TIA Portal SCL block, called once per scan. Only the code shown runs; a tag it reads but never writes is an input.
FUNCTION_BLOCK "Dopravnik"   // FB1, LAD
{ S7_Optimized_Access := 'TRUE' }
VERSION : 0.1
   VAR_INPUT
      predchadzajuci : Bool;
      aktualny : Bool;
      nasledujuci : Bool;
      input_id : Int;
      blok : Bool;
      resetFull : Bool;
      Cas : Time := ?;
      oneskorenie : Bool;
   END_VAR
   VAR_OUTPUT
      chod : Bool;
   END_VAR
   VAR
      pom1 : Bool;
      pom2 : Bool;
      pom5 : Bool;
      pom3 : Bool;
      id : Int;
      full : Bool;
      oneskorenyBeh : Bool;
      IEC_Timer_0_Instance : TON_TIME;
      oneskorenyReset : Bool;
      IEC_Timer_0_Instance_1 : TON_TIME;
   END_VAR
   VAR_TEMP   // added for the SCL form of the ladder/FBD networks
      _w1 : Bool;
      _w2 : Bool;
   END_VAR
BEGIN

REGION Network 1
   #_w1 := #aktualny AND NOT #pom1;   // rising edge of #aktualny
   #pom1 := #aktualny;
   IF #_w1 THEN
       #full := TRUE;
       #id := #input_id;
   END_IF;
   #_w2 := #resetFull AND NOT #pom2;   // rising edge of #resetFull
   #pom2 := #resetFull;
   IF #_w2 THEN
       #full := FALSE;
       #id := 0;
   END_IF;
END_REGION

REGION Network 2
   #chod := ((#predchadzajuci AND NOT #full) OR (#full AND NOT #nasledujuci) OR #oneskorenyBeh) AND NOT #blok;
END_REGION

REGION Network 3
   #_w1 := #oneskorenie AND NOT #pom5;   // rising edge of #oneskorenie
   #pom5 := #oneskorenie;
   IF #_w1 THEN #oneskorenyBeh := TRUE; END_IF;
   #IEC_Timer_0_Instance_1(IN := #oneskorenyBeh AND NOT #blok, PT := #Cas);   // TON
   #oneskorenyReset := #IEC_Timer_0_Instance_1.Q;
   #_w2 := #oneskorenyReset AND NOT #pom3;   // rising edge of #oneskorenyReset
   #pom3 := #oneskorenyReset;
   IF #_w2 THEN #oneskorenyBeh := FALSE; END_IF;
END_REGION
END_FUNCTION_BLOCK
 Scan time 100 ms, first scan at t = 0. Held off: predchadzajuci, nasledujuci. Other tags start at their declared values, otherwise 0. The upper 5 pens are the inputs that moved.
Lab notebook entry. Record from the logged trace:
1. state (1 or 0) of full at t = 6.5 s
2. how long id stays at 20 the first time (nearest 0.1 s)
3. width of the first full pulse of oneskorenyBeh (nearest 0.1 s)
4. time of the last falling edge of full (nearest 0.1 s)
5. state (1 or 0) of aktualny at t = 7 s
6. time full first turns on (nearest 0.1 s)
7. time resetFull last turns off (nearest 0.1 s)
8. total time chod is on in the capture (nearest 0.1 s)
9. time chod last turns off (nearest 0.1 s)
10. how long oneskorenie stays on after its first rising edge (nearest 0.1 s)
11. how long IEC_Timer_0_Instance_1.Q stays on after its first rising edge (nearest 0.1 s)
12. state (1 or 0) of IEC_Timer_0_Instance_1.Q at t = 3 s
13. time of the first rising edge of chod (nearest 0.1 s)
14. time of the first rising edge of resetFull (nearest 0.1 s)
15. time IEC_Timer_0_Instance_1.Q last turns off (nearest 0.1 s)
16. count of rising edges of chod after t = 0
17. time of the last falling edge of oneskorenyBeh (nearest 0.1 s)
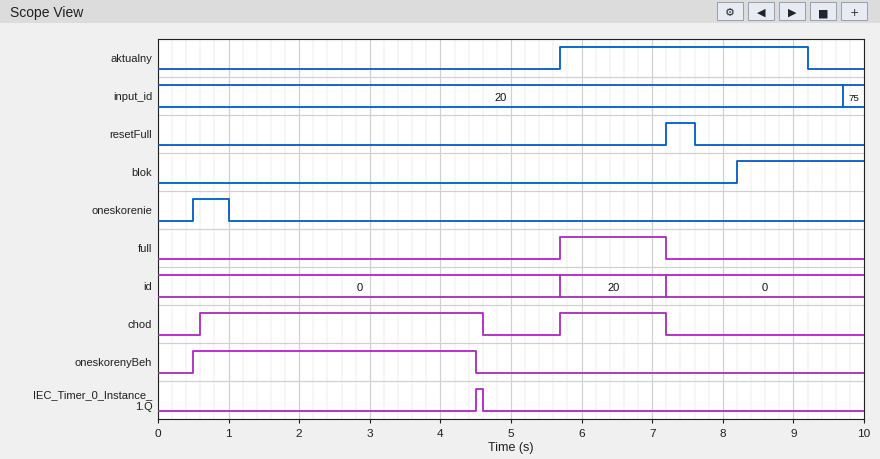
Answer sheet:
1
1.5 s
4.0 s
7.2 s
1
5.7 s
7.6 s
5.5 s
7.2 s
0.5 s
0.1 s
0
0.6 s
7.2 s
4.6 s
2
4.5 s
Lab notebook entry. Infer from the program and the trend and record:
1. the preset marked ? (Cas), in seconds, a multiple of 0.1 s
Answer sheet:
4.0 s
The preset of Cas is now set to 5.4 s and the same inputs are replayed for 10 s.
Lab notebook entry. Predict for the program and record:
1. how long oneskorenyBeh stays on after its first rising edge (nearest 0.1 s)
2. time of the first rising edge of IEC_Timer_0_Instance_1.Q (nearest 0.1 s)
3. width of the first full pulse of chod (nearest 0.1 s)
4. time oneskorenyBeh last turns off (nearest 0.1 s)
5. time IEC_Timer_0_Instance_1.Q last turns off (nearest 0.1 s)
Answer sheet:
5.4 s
5.9 s
6.6 s
5.9 s
6.0 s
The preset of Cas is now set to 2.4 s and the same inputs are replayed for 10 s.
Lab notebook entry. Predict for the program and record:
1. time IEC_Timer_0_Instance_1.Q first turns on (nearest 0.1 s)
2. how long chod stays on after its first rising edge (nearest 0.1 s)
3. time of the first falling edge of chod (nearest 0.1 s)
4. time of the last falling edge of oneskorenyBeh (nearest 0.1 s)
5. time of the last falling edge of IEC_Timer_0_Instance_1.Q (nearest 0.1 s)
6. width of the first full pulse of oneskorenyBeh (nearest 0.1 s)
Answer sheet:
2.9 s
2.4 s
3.0 s
2.9 s
3.0 s
2.4 s
